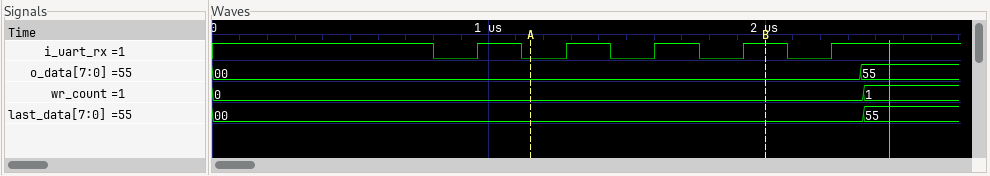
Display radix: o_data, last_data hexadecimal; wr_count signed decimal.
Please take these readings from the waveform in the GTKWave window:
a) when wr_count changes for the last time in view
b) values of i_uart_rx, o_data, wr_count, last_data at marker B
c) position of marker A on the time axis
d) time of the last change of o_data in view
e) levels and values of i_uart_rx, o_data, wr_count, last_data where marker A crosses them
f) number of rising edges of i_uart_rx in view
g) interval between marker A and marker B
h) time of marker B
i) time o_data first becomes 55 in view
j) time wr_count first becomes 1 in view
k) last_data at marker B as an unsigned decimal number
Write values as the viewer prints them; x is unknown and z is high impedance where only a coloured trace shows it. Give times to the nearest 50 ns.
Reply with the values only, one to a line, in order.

2350 ns
i_uart_rx=1, o_data=00, wr_count=0, last_data=00
1150 ns
2350 ns
i_uart_rx=0, o_data=00, wr_count=0, last_data=00
5
850 ns
2000 ns
2350 ns
2350 ns
0
